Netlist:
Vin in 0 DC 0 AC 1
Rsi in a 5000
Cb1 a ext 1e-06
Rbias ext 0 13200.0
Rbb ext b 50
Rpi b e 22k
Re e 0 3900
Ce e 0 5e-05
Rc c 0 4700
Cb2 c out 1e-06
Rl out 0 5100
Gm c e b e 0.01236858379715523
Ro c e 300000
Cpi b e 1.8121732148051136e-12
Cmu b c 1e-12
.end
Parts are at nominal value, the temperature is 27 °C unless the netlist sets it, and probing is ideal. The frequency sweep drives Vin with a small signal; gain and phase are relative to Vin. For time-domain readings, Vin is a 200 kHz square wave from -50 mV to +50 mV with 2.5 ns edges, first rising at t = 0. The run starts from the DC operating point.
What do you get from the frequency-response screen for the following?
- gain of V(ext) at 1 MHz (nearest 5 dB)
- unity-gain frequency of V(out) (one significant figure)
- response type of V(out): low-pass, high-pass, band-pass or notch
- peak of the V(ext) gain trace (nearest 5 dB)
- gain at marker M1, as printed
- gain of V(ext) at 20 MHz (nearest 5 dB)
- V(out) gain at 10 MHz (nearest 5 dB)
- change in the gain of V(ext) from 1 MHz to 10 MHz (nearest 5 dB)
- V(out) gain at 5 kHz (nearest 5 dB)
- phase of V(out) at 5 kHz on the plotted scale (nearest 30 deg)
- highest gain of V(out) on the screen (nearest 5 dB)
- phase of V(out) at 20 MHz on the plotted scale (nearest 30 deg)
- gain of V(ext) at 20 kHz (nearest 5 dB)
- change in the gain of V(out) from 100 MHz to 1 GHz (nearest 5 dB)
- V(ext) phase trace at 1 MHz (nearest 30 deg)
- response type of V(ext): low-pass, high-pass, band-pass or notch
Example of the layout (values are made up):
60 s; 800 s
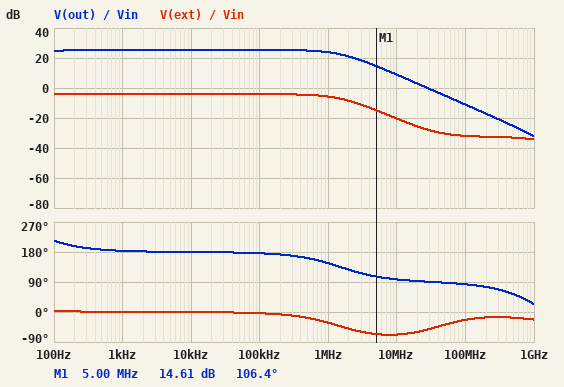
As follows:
-5 dB; 30 MHz; low-pass; -5 dB; 14.61 dB; -25 dB; 10 dB; -15 dB; 25 dB; 180 deg; 25 dB; 90 deg; -5 dB; -20 dB; -30 deg; low-pass
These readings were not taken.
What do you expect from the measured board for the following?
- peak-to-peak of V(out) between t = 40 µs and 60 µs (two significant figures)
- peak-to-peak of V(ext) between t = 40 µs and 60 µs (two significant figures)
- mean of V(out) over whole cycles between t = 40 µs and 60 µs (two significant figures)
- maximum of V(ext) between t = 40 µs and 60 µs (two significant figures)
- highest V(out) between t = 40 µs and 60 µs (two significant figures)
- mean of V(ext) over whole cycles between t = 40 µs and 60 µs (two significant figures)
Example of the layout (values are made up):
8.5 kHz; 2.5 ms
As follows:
1.9 V; 62 mV; -910 mV; 62 mV; 22 mV; 31 mV
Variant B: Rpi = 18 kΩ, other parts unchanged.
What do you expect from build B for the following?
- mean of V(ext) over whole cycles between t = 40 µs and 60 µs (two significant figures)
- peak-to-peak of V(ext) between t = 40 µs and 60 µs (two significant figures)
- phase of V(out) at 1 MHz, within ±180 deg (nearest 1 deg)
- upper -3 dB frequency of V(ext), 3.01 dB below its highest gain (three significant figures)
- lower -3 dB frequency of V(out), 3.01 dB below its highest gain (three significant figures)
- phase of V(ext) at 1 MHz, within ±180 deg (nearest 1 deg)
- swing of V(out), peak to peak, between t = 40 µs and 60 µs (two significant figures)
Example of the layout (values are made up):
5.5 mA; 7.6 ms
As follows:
30 mV; 60 mV; 147 deg; 1.54 MHz; 45.2 Hz; -31 deg; 1.8 V
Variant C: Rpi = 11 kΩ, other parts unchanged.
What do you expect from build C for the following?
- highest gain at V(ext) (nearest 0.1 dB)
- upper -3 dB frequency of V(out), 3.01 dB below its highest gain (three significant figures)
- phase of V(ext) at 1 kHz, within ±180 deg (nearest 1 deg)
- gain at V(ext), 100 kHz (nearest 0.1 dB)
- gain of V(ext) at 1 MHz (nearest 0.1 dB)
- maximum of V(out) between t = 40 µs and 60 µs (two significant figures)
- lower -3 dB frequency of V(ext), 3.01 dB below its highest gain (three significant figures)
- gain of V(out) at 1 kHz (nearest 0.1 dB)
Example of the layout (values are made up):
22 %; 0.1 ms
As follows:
-5.1 dB; 1.72 MHz; 0 deg; -5.3 dB; -6.5 dB; 18 mV; 6.58 Hz; 24.2 dB
